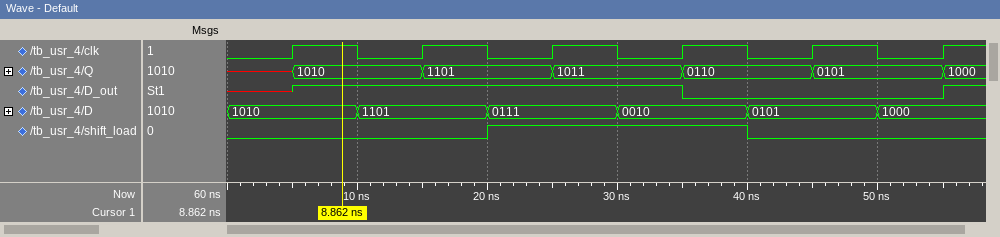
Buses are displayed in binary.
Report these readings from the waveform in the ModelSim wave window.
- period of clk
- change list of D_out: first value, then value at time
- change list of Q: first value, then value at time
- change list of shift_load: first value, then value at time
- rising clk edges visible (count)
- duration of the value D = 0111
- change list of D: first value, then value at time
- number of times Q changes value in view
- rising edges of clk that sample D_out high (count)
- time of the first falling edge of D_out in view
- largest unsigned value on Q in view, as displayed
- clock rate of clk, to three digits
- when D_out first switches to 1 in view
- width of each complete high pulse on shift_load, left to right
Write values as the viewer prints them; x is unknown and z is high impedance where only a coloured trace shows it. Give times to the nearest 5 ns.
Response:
10 ns
x, 1 at 5 ns, 0 at 35 ns, 1 at 55 ns
x, 1010 at 5 ns, 1101 at 15 ns, 1011 at 25 ns, 0110 at 35 ns, 0101 at 45 ns, 1000 at 55 ns
0, 1 at 20 ns, 0 at 40 ns
6
10 ns
1010, 1101 at 10 ns, 0111 at 20 ns, 0010 at 30 ns, 0101 at 40 ns, 1000 at 50 ns
6
3
35 ns
1101
100 MHz
5 ns
20 ns
